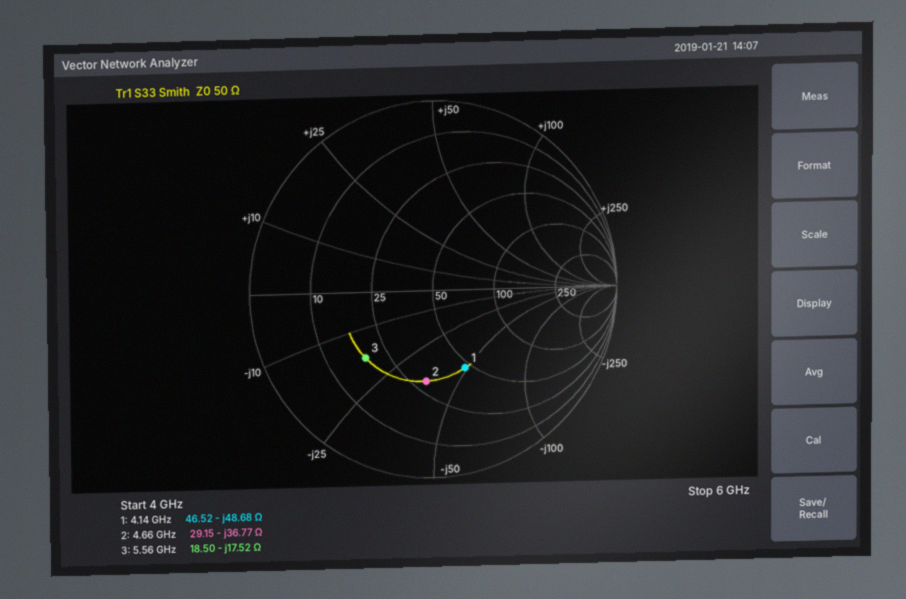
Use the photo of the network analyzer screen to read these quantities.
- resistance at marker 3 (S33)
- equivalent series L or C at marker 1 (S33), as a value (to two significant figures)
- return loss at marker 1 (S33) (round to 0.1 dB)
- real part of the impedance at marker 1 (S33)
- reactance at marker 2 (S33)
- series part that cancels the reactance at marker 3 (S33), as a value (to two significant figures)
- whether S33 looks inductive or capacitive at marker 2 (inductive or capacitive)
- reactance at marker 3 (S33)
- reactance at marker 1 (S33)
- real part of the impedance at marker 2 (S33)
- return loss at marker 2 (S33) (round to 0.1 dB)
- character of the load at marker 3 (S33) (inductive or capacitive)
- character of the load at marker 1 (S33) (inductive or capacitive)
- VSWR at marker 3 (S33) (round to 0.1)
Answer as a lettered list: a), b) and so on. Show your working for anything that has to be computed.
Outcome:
a) 18.50 Ω
b) C = 1/(2π × 4.14 GHz × 48.68 Ω) ≈ 790 fF
c) 6.9 dB
d) 46.52 Ω
e) -36.77 Ω
f) L = 17.52 Ω/(2π × 5.56 GHz) ≈ 502 pH, so 500 pH to two significant figures
g) capacitive
h) -17.52 Ω
i) -48.68 Ω
j) 29.15 Ω
k) 6.3 dB
l) capacitive
m) capacitive
n) 3.1
